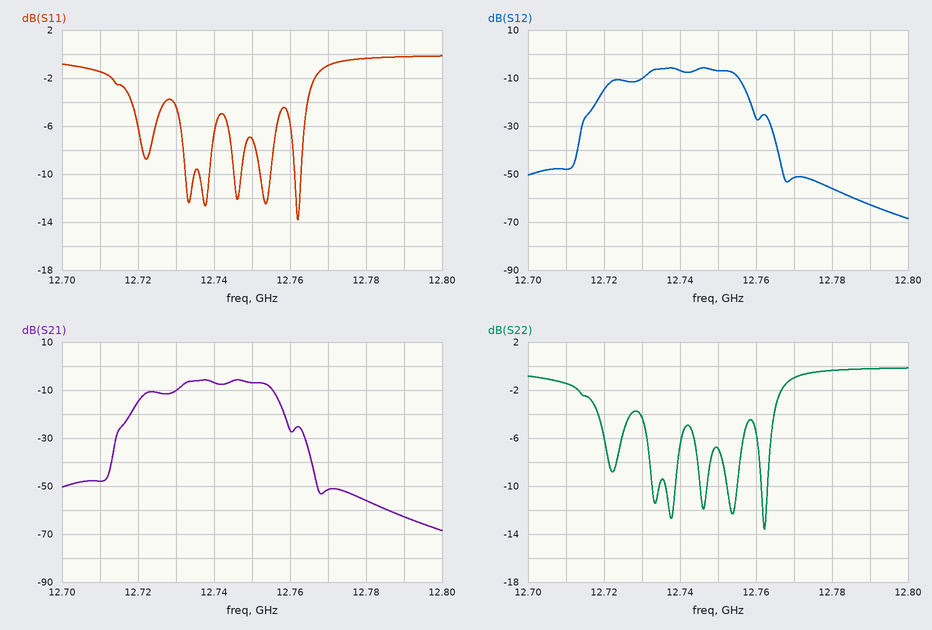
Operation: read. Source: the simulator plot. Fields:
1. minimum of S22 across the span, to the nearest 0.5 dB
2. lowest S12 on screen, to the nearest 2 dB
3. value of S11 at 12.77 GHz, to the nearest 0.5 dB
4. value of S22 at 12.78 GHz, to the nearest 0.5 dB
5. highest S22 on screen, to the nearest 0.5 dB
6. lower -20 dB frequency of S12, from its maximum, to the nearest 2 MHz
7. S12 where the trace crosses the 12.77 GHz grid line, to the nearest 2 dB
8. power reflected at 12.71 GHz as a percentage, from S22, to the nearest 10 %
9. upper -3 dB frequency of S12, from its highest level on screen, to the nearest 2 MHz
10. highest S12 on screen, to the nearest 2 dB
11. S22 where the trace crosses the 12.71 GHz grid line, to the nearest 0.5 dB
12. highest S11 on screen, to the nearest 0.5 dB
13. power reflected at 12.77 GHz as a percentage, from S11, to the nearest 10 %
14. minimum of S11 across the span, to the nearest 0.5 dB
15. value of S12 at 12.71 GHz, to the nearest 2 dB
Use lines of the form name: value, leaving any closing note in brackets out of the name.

minimum of S22 across the span, to the nearest 0.5 dB: -13.5 dB
lowest S12 on screen, to the nearest 2 dB: -68 dB
value of S11 at 12.77 GHz, to the nearest 0.5 dB: -1.0 dB
value of S22 at 12.78 GHz, to the nearest 0.5 dB: -0.5 dB
highest S22 on screen, to the nearest 0.5 dB: 0.0 dB
lower -20 dB frequency of S12, from its maximum, to the nearest 2 MHz: 12.716 GHz
S12 where the trace crosses the 12.77 GHz grid line, to the nearest 2 dB: -52 dB
power reflected at 12.71 GHz as a percentage, from S22, to the nearest 10 %: 70 %
upper -3 dB frequency of S12, from its highest level on screen, to the nearest 2 MHz: 12.754 GHz
highest S12 on screen, to the nearest 2 dB: -6 dB
S22 where the trace crosses the 12.71 GHz grid line, to the nearest 0.5 dB: -1.5 dB
highest S11 on screen, to the nearest 0.5 dB: 0.0 dB
power reflected at 12.77 GHz as a percentage, from S11, to the nearest 10 %: 80 %
minimum of S11 across the span, to the nearest 0.5 dB: -14.0 dB
value of S12 at 12.71 GHz, to the nearest 2 dB: -48 dB
